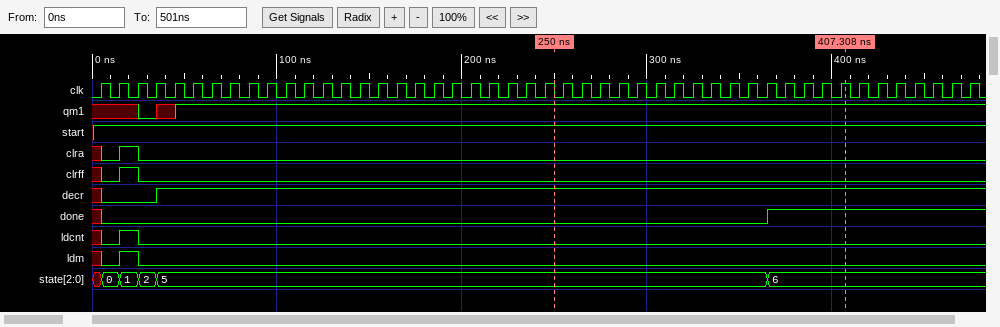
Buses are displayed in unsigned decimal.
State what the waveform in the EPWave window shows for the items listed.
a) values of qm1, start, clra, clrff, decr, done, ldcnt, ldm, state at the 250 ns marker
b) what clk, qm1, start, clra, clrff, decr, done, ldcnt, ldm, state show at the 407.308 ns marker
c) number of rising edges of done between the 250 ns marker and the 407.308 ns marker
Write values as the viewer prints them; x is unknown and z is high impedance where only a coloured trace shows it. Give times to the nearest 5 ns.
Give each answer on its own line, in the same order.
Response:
qm1=1, start=1, clra=0, clrff=0, decr=1, done=0, ldcnt=0, ldm=0, state=5
clk=1, qm1=1, start=1, clra=0, clrff=0, decr=1, done=1, ldcnt=0, ldm=0, state=6
1
